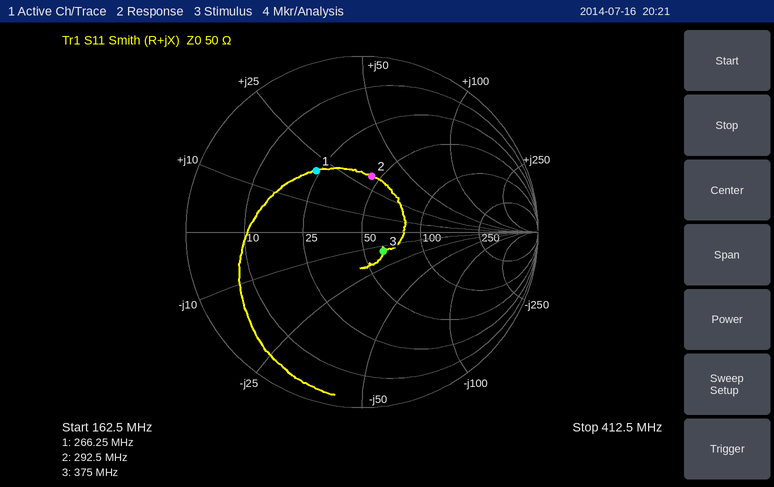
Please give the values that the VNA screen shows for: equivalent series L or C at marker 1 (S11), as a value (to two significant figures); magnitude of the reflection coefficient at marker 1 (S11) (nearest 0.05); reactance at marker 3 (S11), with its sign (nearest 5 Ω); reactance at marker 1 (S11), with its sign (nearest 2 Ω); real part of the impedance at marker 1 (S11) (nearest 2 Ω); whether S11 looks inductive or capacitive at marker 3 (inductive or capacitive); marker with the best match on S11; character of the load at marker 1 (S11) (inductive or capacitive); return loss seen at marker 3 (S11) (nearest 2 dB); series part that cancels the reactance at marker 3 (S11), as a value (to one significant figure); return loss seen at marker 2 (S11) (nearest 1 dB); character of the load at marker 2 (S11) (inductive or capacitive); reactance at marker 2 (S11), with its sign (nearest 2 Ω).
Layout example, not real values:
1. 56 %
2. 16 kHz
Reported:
1. 12 nH
2. 0.45
3. -15 Ω
4. +20 Ω
5. 24 Ω
6. capacitive
7. marker 3
8. inductive
9. 16 dB
10. 6 nH
11. 10 dB
12. inductive
13. +32 Ω
